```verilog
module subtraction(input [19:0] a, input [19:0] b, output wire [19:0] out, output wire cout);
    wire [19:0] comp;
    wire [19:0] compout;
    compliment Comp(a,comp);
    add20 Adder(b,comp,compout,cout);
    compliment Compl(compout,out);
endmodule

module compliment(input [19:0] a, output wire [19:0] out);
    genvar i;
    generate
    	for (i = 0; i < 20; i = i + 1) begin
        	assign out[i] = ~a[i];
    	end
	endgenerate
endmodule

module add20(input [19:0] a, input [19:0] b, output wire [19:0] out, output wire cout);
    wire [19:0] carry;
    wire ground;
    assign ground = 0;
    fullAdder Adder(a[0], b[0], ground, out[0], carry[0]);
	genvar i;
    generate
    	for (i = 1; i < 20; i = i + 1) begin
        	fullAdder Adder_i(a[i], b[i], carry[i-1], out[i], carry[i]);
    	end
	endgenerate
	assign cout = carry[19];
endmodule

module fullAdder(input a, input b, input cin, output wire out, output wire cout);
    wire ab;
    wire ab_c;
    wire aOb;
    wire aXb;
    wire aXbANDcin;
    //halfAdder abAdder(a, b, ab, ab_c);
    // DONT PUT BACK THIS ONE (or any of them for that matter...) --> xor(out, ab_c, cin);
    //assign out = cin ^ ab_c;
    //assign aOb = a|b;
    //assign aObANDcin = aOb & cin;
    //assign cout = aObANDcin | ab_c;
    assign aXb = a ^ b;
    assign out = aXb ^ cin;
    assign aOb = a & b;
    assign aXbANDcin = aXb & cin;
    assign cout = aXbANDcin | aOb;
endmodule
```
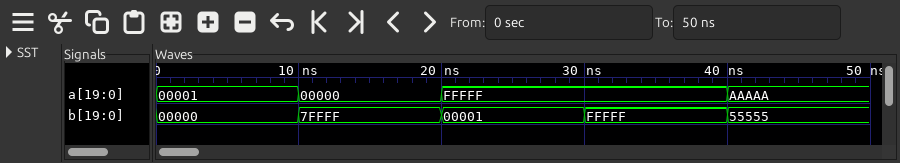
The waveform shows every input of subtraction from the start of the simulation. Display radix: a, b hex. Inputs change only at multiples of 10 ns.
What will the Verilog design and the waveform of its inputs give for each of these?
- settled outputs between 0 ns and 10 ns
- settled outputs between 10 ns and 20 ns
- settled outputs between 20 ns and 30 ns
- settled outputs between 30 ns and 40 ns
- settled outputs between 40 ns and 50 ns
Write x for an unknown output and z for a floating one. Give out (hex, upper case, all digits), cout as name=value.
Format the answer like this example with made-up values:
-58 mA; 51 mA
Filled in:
out=00001, cout=0; out=80001, cout=1; out=FFFFE, cout=0; out=00000, cout=0; out=55555, cout=0
